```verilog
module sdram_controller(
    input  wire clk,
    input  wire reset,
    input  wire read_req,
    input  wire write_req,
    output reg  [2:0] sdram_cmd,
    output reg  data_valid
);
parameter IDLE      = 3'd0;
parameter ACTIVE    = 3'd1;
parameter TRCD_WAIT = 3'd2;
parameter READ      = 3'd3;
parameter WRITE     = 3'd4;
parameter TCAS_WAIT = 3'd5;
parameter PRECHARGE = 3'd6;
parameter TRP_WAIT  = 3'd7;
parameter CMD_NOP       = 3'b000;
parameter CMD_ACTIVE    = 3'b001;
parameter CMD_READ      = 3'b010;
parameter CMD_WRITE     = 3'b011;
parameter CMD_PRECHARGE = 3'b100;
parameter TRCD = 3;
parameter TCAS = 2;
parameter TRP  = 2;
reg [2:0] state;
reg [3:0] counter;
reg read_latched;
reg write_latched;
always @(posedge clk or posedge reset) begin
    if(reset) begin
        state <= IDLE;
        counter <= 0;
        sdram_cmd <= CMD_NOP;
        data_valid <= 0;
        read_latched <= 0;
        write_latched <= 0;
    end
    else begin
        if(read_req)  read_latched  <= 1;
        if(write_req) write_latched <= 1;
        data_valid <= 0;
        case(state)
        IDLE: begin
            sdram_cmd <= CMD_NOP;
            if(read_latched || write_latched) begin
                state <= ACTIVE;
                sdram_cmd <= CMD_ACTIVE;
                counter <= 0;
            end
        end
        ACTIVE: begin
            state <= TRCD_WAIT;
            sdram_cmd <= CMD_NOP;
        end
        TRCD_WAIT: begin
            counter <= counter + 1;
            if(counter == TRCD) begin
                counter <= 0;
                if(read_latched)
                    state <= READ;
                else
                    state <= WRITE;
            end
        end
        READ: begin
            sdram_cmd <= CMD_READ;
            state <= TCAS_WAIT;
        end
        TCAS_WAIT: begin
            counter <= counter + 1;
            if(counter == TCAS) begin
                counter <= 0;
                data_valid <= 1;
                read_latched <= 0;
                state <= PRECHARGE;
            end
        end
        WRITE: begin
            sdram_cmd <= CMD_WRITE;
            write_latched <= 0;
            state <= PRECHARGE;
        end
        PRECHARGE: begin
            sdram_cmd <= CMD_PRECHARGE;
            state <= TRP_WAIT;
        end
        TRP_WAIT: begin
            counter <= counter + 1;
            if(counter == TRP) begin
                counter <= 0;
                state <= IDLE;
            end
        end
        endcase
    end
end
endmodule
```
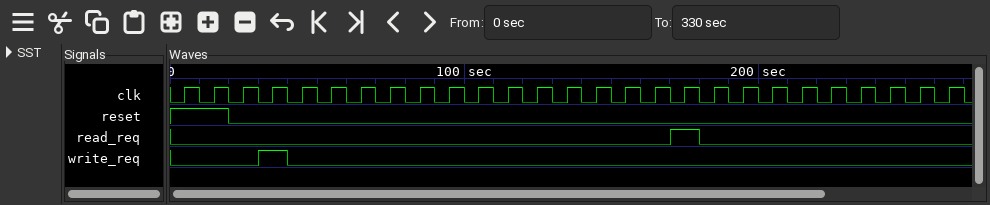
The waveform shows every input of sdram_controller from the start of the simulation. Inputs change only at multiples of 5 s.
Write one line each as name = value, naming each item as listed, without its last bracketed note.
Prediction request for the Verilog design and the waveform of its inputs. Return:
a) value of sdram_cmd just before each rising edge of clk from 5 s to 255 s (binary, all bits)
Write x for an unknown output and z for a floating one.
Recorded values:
value of sdram_cmd just before each rising edge of clk from 5 s to 255 s = 000, 000, 000, 000, 000, 001, 000, 000, 000, 000, 000, 011, 100, 100, 100, 100, 000, 000, 000, 001, 000, 000, 000, 000, 000, 010
